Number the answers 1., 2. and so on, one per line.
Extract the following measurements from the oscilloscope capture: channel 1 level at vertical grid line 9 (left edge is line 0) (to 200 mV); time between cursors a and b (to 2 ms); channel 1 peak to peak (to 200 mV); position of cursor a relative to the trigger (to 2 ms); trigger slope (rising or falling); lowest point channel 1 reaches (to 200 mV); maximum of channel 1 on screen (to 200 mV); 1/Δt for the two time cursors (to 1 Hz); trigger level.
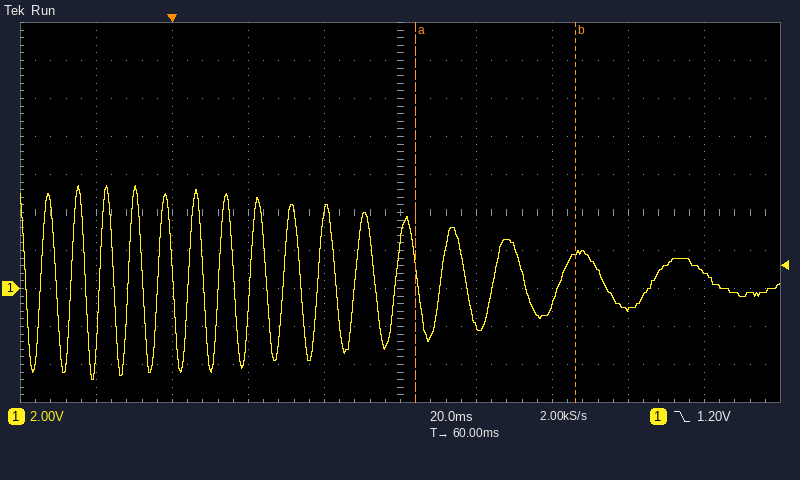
1. 800 mV
2. 42 ms
3. 10.2 V
4. +64 ms
5. falling
6. -4.8 V
7. 5.4 V
8. 24 Hz
9. 1.20 V
